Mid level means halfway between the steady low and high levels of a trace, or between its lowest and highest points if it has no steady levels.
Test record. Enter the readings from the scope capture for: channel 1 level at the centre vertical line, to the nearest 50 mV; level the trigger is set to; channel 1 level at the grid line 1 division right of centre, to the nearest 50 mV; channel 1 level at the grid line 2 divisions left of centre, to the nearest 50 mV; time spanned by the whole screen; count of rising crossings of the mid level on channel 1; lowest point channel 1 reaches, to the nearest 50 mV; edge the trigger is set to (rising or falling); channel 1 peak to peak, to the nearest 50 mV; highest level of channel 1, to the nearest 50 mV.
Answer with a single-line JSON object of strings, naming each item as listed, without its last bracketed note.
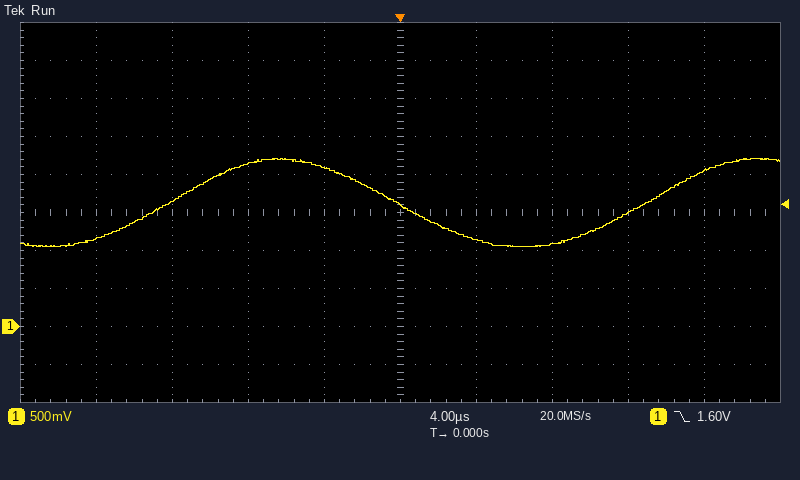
{"channel 1 level at the centre vertical line, to the nearest 50 mV": "1.60 V", "level the trigger is set to": "1.60 V", "channel 1 level at the grid line 1 division right of centre, to the nearest 50 mV": "1.15 V", "channel 1 level at the grid line 2 divisions left of centre, to the nearest 50 mV": "2.15 V", "time spanned by the whole screen": "40 µs", "count of rising crossings of the mid level on channel 1": "2", "lowest point channel 1 reaches, to the nearest 50 mV": "1.05 V", "edge the trigger is set to": "falling", "channel 1 peak to peak, to the nearest 50 mV": "1.15 V", "highest level of channel 1, to the nearest 50 mV": "2.20 V"}
